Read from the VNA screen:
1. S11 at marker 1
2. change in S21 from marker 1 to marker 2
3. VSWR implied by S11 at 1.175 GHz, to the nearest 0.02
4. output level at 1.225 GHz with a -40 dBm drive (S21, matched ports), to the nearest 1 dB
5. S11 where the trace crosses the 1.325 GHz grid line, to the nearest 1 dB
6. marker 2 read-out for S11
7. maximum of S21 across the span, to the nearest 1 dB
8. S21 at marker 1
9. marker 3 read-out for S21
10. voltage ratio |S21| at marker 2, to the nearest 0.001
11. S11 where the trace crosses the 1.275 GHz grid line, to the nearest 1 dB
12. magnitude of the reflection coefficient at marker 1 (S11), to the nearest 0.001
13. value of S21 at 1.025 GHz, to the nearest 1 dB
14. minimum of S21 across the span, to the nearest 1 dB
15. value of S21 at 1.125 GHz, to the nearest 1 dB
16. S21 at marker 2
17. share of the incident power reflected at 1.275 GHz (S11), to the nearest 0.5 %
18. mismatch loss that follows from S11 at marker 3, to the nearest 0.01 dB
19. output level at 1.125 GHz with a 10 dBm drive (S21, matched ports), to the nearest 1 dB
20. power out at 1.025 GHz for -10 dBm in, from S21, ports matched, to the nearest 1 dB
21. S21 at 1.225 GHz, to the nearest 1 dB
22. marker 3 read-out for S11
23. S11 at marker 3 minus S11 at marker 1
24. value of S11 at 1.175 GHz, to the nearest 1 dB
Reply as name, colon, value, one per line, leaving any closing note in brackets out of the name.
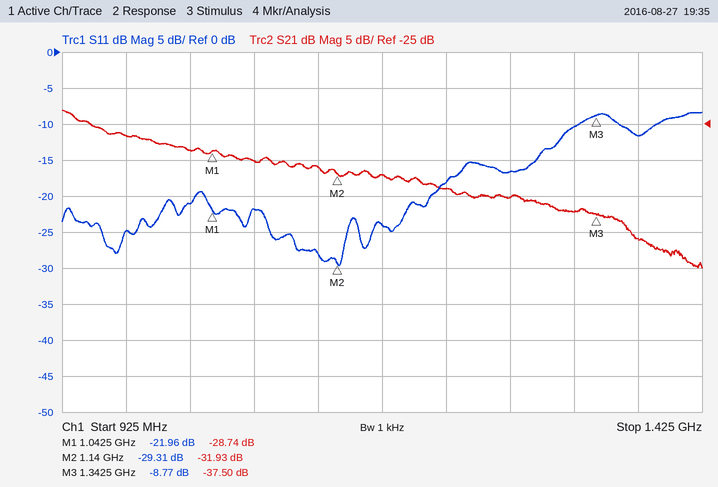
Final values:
S11 at marker 1: -21.96 dB
change in S21 from marker 1 to marker 2: -3.19 dB
VSWR implied by S11 at 1.175 GHz, to the nearest 0.02: 1.14
output level at 1.225 GHz with a -40 dBm drive (S21, matched ports), to the nearest 1 dB: -74 dBm
S11 where the trace crosses the 1.325 GHz grid line, to the nearest 1 dB: -10 dB
marker 2 read-out for S11: -29.31 dB
maximum of S21 across the span, to the nearest 1 dB: -23 dB
S21 at marker 1: -28.74 dB
marker 3 read-out for S21: -37.50 dB
voltage ratio |S21| at marker 2, to the nearest 0.001: 0.025
S11 where the trace crosses the 1.275 GHz grid line, to the nearest 1 dB: -17 dB
magnitude of the reflection coefficient at marker 1 (S11), to the nearest 0.001: 0.080
value of S21 at 1.025 GHz, to the nearest 1 dB: -29 dB
minimum of S21 across the span, to the nearest 1 dB: -45 dB
value of S21 at 1.125 GHz, to the nearest 1 dB: -31 dB
S21 at marker 2: -31.93 dB
share of the incident power reflected at 1.275 GHz (S11), to the nearest 0.5 %: 2.0 %
mismatch loss that follows from S11 at marker 3, to the nearest 0.01 dB: 0.62 dB
output level at 1.125 GHz with a 10 dBm drive (S21, matched ports), to the nearest 1 dB: -21 dBm
power out at 1.025 GHz for -10 dBm in, from S21, ports matched, to the nearest 1 dB: -39 dBm
S21 at 1.225 GHz, to the nearest 1 dB: -34 dB
marker 3 read-out for S11: -8.77 dB
S11 at marker 3 minus S11 at marker 1: 13.19 dB
value of S11 at 1.175 GHz, to the nearest 1 dB: -24 dB
